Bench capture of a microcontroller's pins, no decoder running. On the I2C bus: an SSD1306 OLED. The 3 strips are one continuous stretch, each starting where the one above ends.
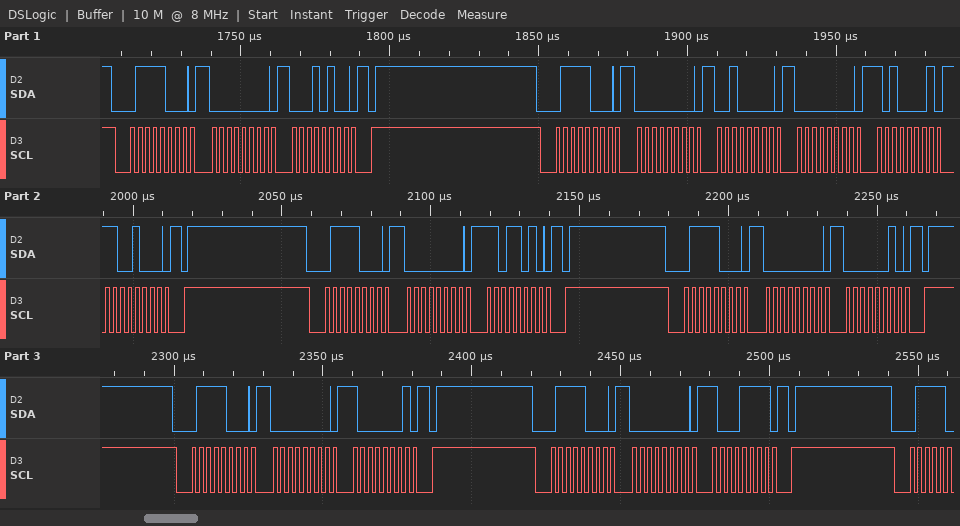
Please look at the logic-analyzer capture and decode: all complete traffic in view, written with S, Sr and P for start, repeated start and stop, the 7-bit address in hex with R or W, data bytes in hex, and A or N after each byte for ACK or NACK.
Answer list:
S 3CW A 00 A 14 A P S 3CW A 00 A 20 A 00 A A1 A C8 A P S 3CW A 00 A DA A P S 3CW A 00 A 02 A P S 3CW A 00 A 81 A P S 3CW A 00 A 8F A P
